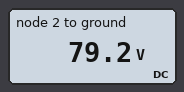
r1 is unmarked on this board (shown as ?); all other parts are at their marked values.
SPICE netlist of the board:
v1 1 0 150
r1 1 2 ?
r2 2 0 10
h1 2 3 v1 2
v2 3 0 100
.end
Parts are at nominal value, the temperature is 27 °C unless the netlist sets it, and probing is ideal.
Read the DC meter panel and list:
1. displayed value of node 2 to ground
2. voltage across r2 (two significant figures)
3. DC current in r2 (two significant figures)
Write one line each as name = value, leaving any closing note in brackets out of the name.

displayed value of node 2 to ground = 79.2 V
voltage across r2 = 79 V
DC current in r2 = 7.9 A
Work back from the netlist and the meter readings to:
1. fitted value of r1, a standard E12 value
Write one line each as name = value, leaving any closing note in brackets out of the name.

fitted value of r1, a standard E12 value = 6.8 Ω
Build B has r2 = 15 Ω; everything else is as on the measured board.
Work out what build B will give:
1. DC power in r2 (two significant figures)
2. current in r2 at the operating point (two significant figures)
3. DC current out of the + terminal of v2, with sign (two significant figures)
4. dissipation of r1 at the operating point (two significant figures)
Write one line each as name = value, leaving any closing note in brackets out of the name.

DC power in r2 = 420 W
current in r2 at the operating point = 5.3 A
DC current out of the + terminal of v2, with sign = -5.1 A
dissipation of r1 at the operating point = 740 W
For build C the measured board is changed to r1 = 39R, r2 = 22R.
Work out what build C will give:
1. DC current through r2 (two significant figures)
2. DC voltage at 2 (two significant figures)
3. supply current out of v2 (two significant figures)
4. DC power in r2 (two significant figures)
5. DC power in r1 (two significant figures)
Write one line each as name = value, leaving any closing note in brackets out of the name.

DC current through r2 = 4.4 A
DC voltage at 2 = 97 V
supply current out of v2 = 3.1 A
DC power in r2 = 430 W
DC power in r1 = 71 W
